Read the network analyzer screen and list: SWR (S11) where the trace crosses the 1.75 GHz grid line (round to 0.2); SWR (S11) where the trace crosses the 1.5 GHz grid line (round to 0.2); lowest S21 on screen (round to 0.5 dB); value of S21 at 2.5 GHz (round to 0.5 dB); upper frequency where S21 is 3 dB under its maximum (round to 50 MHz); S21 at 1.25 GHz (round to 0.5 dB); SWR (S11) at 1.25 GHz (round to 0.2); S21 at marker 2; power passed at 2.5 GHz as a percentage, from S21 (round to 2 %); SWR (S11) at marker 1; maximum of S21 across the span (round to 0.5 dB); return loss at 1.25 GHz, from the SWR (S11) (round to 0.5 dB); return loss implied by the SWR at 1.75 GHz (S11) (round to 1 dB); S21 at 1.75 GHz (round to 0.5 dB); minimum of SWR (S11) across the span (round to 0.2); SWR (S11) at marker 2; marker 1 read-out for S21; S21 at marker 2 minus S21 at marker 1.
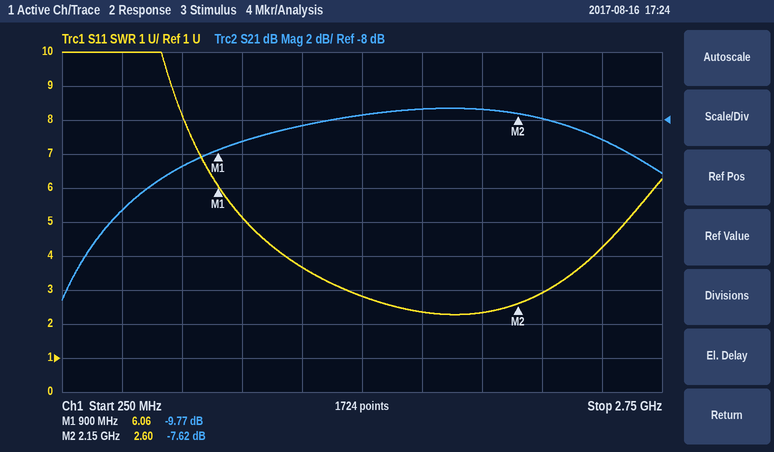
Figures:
2.4
2.8
-18.5 dB
-9.0 dB
2.65 GHz
-8.5 dB
3.6
-7.62 dB
12 %
6.06
-7.5 dB
5.0 dB
8 dB
-7.5 dB
2.2
2.60
-9.77 dB
2.15 dB
